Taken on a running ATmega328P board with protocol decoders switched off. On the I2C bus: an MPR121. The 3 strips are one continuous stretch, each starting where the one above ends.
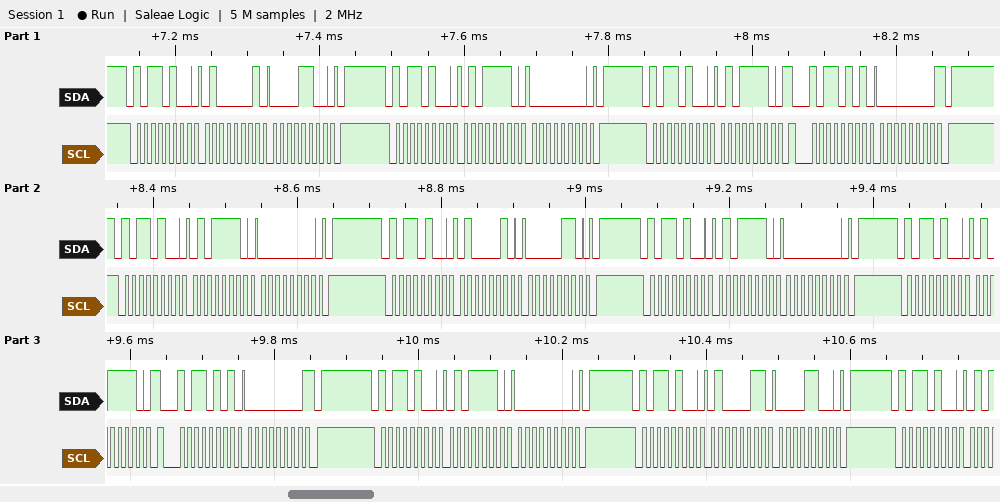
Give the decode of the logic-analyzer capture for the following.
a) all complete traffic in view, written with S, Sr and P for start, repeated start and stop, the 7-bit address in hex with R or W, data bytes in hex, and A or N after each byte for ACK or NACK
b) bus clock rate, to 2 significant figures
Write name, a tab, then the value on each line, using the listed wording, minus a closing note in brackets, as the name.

all complete traffic in view, written with S, Sr and P for start, repeated start and stop, the 7-bit address in hex with R or W, data bytes in hex, and A or N after each byte for ACK or NACK	S 5AW A 41 A 0C A P S 5AW A 5E A 00 A P S 5AW A 5E A Sr 5AR A 00 N P S 5AW A 5E A 00 A P S 5AW A 42 A 06 A P S 5AW A 5E A 00 A P S 5AW A 5E A Sr 5AR A 00 N P S 5AW A 5E A 00 A P S 5AW A 43 A 0C A P S 5AW A
bus clock rate, to 2 significant figures	100 kHz
